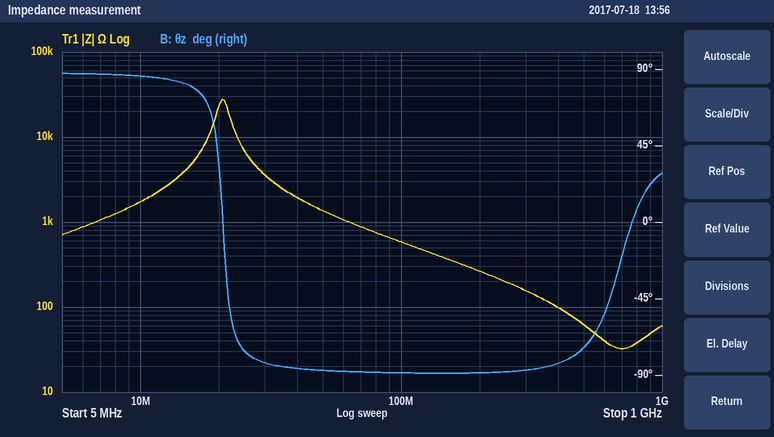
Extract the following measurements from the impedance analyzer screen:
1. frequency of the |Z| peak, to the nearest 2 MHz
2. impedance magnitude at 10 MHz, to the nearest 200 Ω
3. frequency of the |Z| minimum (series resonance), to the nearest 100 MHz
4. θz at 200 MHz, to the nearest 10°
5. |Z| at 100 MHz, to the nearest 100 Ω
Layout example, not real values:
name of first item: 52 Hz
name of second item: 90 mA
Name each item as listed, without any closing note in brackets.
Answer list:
frequency of the |Z| peak, to the nearest 2 MHz: 20 MHz
impedance magnitude at 10 MHz, to the nearest 200 Ω: 1.8 kΩ
frequency of the |Z| minimum (series resonance), to the nearest 100 MHz: 700 MHz
θz at 200 MHz, to the nearest 10°: -90°
|Z| at 100 MHz, to the nearest 100 Ω: 600 Ω
